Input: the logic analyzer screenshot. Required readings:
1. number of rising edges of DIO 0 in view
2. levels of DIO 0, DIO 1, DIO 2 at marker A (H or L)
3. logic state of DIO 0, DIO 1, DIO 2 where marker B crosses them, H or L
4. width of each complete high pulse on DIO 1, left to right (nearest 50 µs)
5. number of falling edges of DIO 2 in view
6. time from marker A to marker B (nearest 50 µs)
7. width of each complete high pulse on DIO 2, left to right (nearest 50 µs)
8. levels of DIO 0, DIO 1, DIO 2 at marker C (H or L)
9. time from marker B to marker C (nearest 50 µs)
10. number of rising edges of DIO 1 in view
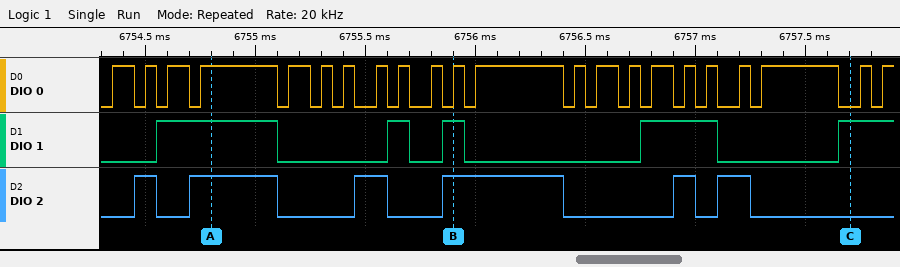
22
DIO 0=H, DIO 1=H, DIO 2=H
DIO 0=H, DIO 1=H, DIO 2=H
550 µs, 100 µs, 100 µs, 350 µs
6
1100 µs
100 µs, 400 µs, 150 µs, 550 µs, 100 µs, 150 µs
DIO 0=L, DIO 1=H, DIO 2=L
1800 µs
5
